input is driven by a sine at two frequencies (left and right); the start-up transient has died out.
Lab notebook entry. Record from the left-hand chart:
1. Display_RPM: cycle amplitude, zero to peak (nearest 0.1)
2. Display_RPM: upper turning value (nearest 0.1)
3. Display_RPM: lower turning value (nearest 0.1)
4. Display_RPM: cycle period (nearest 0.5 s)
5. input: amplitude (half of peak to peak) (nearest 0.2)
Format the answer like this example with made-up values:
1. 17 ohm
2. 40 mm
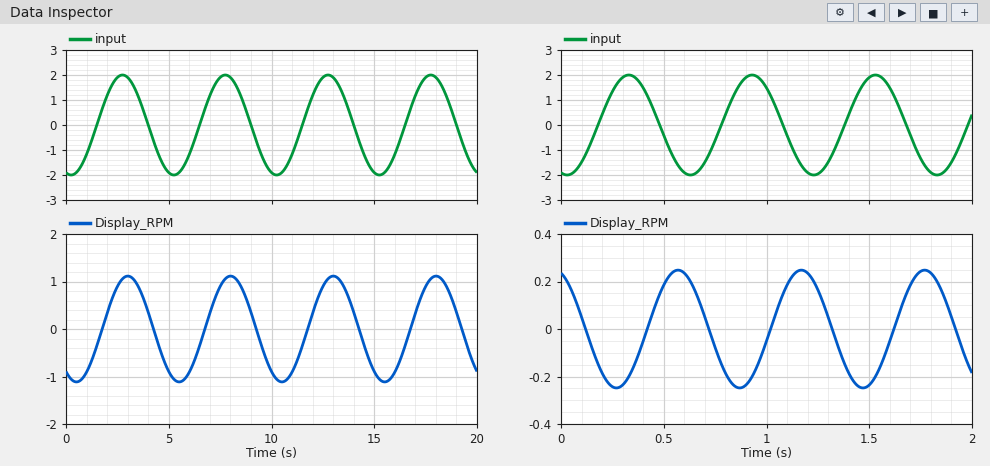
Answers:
1. 1.1
2. 1.1
3. -1.1
4. 5.0 s
5. 2.0
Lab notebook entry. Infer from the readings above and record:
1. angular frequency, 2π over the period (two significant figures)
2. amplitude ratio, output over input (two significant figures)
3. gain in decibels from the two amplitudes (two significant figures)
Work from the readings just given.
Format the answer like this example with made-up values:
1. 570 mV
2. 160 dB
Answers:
1. 1.3 rad/s
2. 0.55
3. -5.2 dB
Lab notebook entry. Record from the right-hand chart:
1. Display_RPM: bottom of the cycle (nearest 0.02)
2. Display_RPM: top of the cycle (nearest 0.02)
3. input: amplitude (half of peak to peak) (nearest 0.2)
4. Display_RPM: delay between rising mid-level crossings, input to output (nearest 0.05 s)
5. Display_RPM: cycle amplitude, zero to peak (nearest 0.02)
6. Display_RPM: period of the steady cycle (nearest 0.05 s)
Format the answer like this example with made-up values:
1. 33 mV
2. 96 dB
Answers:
1. -0.24
2. 0.24
3. 2.0
4. 0.25 s
5. 0.24
6. 0.60 s
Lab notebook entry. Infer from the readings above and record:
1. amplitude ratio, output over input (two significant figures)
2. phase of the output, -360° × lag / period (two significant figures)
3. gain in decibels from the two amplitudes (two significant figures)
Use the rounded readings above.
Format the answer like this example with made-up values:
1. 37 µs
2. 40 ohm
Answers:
1. 0.12
2. -150°
3. -18 dB
